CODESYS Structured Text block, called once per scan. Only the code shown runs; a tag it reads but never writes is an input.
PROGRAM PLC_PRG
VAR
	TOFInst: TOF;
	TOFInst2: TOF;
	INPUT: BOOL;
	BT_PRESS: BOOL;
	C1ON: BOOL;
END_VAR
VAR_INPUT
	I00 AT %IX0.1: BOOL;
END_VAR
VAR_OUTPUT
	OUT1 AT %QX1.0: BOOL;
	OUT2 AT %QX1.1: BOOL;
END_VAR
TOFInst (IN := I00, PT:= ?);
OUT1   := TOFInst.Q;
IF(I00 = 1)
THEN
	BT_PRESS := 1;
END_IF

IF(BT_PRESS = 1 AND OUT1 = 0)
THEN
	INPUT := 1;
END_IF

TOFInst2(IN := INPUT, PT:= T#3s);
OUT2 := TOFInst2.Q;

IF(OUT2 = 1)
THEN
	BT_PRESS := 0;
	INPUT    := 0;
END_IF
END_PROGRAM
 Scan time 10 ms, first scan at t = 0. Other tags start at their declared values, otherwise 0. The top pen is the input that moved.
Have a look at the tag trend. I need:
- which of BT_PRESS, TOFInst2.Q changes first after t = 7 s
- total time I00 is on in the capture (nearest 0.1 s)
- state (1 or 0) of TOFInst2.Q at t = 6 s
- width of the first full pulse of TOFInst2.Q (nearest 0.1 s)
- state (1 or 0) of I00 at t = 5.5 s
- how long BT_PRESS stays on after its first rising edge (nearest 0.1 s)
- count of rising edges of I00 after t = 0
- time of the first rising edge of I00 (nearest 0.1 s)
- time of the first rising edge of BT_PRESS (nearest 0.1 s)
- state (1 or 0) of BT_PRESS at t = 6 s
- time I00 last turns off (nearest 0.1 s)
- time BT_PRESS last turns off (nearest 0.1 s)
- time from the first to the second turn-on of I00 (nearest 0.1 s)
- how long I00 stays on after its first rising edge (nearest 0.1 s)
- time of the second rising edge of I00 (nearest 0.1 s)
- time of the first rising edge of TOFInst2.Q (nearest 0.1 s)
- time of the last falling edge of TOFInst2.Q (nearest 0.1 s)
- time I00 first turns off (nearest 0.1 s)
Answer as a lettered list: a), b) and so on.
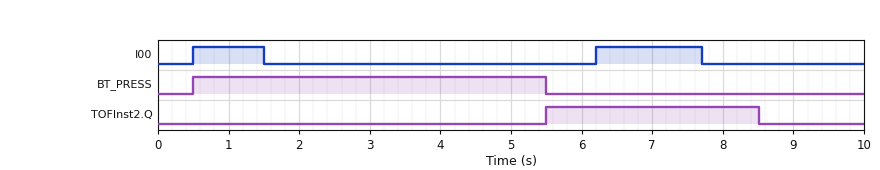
a) TOFInst2.Q
b) 2.5 s
c) 1
d) 3.0 s
e) 0
f) 5.0 s
g) 2
h) 0.5 s
i) 0.5 s
j) 0
k) 7.7 s
l) 5.5 s
m) 5.7 s
n) 1.0 s
o) 6.2 s
p) 5.5 s
q) 8.5 s
r) 1.5 s
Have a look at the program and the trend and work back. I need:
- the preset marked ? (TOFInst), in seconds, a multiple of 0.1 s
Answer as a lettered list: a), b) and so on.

a) 4.0 s
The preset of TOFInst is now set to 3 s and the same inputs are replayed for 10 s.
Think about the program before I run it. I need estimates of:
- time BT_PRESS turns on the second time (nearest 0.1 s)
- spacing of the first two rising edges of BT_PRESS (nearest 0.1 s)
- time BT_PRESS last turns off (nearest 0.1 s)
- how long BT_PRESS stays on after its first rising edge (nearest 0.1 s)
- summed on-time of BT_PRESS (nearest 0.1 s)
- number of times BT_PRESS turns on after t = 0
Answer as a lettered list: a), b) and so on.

a) 7.5 s
b) 7.0 s
c) 4.5 s
d) 4.0 s
e) 6.5 s
f) 2
